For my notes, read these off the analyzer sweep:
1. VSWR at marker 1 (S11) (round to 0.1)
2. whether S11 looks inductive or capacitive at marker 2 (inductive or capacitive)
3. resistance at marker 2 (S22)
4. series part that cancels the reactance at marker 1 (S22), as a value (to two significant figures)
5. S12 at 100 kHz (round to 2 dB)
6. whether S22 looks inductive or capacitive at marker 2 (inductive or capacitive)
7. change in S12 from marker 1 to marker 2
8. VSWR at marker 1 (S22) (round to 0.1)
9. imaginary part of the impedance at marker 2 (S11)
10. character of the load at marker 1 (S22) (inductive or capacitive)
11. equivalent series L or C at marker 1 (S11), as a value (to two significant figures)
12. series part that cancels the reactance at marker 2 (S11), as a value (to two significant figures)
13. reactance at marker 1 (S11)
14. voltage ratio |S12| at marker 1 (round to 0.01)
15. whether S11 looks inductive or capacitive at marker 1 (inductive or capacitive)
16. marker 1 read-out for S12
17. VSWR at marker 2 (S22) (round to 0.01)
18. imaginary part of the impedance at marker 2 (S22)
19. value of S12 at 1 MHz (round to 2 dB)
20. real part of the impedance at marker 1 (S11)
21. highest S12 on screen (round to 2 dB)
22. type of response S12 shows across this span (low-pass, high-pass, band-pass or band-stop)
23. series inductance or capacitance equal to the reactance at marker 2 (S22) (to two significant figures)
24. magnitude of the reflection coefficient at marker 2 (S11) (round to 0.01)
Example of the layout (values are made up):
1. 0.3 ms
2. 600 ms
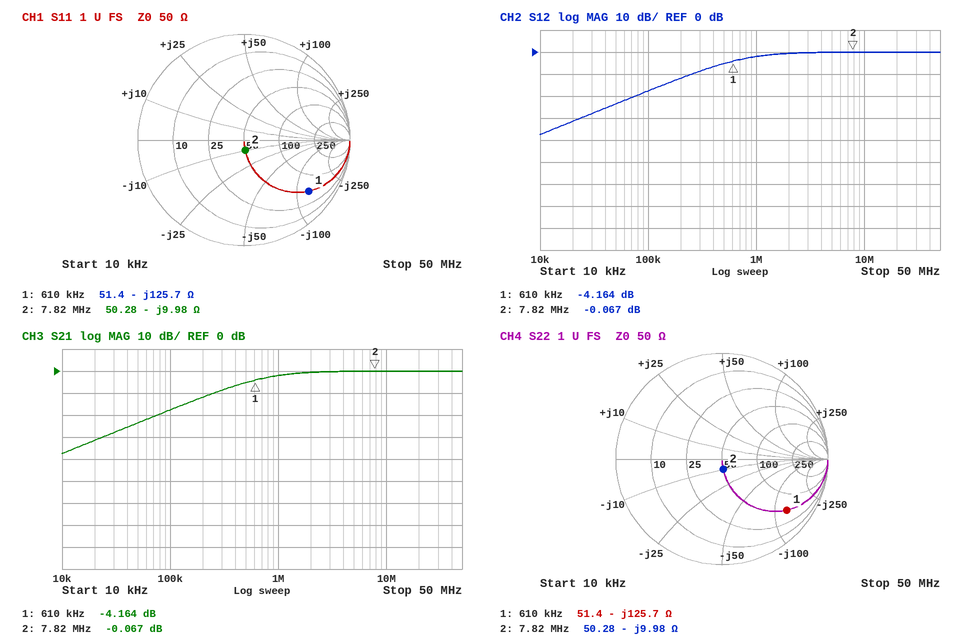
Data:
1. 8.0
2. capacitive
3. 50.28 Ω
4. 33 µH
5. -18 dB
6. capacitive
7. 4.097 dB
8. 8.0
9. -9.98 Ω
10. capacitive
11. 2.1 nF
12. 200 nH
13. -125.7 Ω
14. 0.62
15. capacitive
16. -4.164 dB
17. 1.22
18. -9.98 Ω
19. -2 dB
20. 51.4 Ω
21. 0 dB
22. high-pass
23. 2.0 nF
24. 0.10
